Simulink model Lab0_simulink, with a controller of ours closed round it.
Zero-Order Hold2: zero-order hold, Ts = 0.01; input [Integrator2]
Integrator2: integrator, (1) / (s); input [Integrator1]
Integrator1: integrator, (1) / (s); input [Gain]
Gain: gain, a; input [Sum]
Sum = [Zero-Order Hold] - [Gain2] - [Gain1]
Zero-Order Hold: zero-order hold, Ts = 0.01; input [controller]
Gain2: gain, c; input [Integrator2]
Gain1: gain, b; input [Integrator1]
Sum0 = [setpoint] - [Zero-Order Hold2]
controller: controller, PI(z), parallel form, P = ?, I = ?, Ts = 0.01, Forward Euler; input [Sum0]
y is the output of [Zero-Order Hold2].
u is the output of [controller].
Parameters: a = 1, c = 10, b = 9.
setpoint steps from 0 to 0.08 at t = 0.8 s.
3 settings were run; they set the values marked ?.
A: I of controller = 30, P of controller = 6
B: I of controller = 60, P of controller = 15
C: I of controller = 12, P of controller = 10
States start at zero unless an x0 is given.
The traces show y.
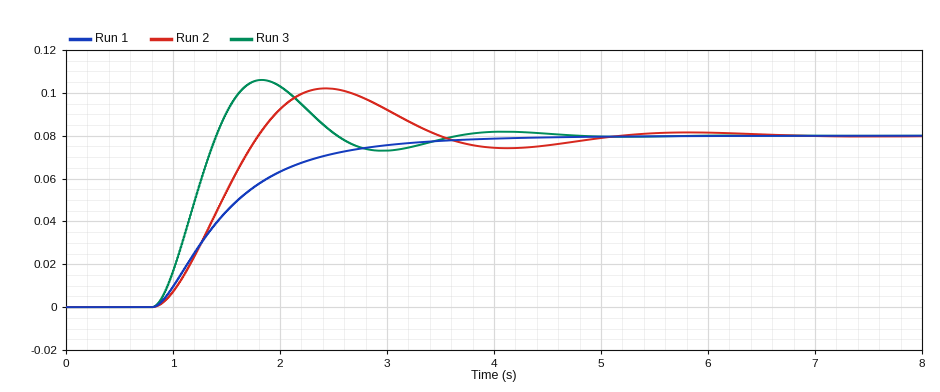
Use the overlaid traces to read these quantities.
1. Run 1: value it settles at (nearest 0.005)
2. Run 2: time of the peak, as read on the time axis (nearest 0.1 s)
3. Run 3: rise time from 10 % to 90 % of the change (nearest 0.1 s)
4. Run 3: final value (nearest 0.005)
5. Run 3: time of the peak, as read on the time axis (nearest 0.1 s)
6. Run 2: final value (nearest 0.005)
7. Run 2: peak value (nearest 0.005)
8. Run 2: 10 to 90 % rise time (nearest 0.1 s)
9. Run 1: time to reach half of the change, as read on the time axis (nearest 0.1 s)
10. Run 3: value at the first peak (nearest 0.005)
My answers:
0.080
2.4 s
0.4 s
0.080
1.8 s
0.080
0.100
0.7 s
1.4 s
0.105
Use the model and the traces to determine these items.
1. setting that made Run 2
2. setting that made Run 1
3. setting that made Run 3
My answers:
A
C
B
